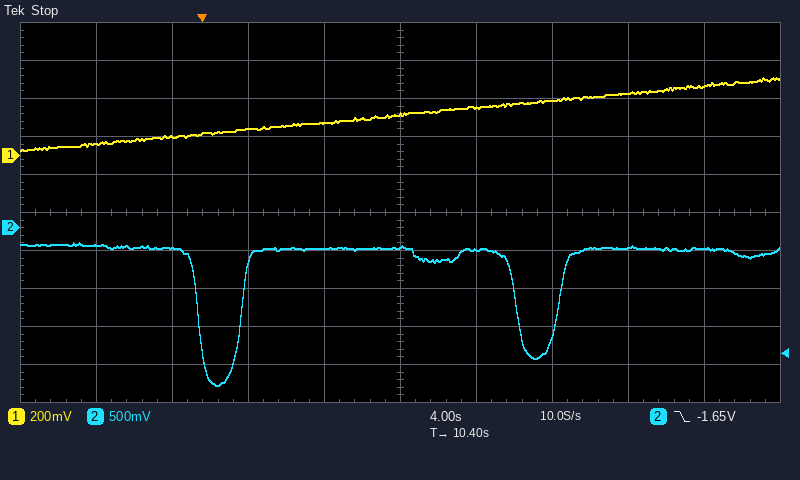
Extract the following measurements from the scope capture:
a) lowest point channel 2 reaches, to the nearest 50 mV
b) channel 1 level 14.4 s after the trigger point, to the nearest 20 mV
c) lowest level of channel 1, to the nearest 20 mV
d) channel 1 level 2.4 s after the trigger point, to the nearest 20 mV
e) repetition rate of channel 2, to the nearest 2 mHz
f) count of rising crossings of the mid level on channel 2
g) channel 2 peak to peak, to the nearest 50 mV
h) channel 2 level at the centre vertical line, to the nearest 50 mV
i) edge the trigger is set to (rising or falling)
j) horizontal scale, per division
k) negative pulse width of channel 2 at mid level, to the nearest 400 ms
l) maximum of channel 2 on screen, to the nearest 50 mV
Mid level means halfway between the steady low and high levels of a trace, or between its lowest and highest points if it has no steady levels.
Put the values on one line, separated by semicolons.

-2.10 V; 260 mV; 20 mV; 140 mV; 60 mHz; 2; 1.90 V; -250 mV; falling; 4 s; 2.0 s; -200 mV
